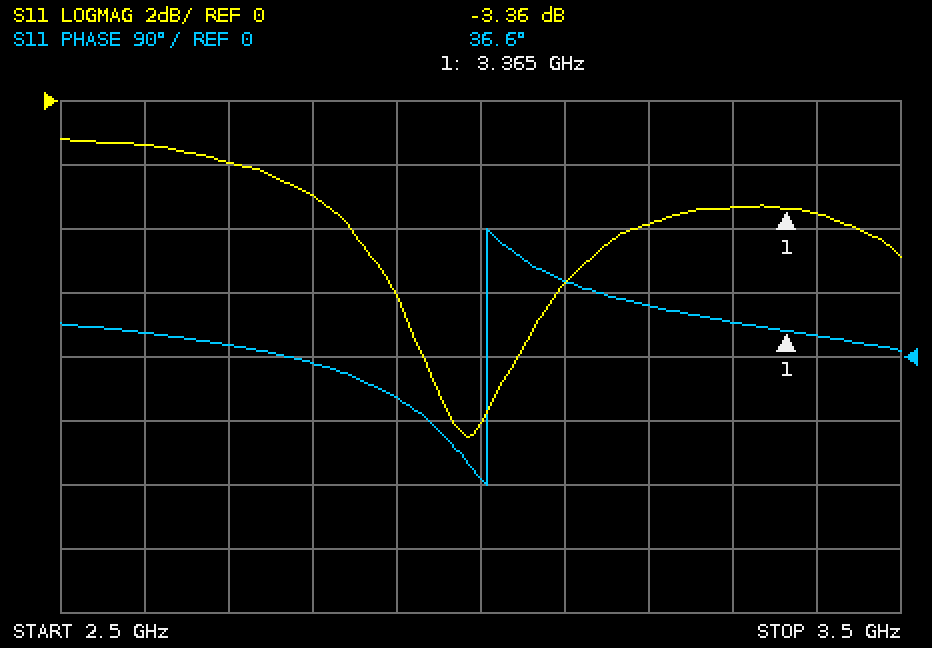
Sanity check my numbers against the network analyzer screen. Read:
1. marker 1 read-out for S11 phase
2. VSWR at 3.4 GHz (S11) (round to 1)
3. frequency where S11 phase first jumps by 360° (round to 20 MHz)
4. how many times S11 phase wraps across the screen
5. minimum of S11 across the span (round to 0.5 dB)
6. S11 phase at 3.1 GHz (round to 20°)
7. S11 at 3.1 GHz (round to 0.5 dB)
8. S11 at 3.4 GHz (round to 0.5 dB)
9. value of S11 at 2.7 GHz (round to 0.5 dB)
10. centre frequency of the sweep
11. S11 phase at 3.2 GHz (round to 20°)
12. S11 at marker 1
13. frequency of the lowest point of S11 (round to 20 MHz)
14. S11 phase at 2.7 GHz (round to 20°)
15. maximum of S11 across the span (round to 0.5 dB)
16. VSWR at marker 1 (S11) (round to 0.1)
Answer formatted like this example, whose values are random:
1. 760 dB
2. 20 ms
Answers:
1. 36.6°
2. 5
3. 3.00 GHz
4. 1
5. -10.5 dB
6. 100°
7. -5.5 dB
8. -3.5 dB
9. -2.0 dB
10. 3 GHz
11. 80°
12. -3.36 dB
13. 2.98 GHz
14. 20°
15. -1.0 dB
16. 5.2
